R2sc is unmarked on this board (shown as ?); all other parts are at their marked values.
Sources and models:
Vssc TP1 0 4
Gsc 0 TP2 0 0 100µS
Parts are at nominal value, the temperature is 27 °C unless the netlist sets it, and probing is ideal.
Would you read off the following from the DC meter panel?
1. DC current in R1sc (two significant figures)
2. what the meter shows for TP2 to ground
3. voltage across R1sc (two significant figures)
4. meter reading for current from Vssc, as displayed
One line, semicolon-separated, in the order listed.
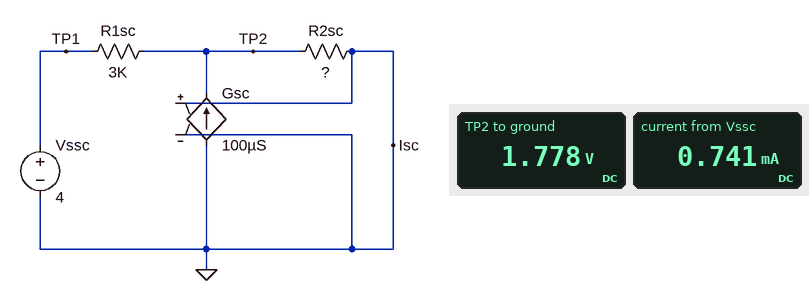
740 µA; 1.778 V; 2.2 V; 0.741 mA
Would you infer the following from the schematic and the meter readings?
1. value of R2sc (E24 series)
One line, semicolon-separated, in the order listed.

2.4 kΩ
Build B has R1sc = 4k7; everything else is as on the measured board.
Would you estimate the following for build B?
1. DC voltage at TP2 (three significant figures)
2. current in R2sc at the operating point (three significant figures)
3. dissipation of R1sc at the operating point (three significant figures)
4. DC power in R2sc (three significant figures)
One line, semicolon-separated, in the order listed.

1.35 V; 563 µA; 1.49 mW; 762 µW
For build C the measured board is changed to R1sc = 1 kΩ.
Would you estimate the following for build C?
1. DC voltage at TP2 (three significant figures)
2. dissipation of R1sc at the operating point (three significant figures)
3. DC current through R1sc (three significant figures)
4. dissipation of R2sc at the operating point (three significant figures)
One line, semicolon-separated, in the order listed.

2.82 V; 1.38 mW; 1.18 mA; 3.32 mW
